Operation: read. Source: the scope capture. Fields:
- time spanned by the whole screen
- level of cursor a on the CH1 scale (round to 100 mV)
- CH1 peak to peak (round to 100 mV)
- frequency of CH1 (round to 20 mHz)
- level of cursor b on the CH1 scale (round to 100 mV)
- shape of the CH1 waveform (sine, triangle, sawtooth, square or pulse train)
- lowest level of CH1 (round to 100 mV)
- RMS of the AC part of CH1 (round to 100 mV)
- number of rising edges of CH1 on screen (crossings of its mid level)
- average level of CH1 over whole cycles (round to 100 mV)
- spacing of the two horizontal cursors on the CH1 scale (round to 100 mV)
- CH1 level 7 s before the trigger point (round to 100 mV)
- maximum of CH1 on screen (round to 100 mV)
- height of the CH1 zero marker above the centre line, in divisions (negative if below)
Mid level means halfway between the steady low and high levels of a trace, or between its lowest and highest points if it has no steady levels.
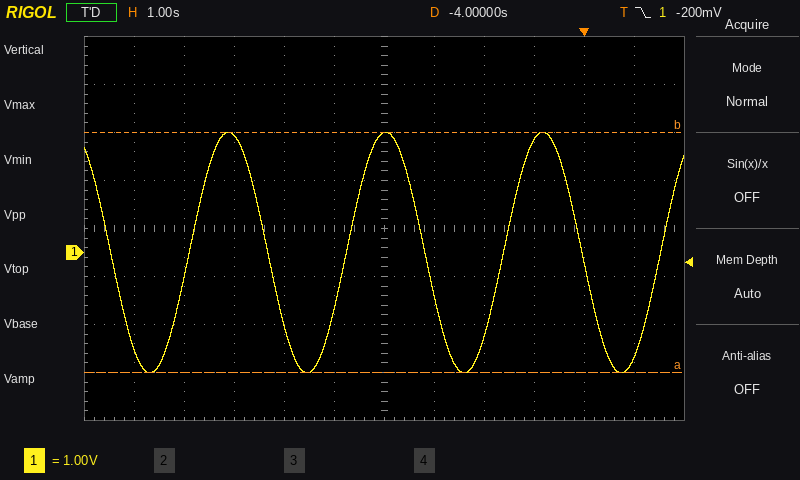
12 s
-2.5 V
5.0 V
320 mHz
2.5 V
sine
-2.5 V
1.8 V
4
0.0 V
5.0 V
2.4 V
2.5 V
-0.5 div
